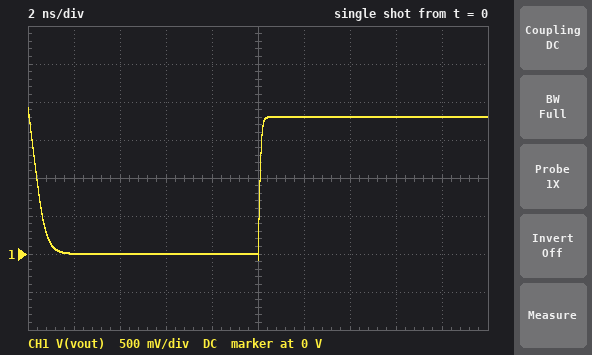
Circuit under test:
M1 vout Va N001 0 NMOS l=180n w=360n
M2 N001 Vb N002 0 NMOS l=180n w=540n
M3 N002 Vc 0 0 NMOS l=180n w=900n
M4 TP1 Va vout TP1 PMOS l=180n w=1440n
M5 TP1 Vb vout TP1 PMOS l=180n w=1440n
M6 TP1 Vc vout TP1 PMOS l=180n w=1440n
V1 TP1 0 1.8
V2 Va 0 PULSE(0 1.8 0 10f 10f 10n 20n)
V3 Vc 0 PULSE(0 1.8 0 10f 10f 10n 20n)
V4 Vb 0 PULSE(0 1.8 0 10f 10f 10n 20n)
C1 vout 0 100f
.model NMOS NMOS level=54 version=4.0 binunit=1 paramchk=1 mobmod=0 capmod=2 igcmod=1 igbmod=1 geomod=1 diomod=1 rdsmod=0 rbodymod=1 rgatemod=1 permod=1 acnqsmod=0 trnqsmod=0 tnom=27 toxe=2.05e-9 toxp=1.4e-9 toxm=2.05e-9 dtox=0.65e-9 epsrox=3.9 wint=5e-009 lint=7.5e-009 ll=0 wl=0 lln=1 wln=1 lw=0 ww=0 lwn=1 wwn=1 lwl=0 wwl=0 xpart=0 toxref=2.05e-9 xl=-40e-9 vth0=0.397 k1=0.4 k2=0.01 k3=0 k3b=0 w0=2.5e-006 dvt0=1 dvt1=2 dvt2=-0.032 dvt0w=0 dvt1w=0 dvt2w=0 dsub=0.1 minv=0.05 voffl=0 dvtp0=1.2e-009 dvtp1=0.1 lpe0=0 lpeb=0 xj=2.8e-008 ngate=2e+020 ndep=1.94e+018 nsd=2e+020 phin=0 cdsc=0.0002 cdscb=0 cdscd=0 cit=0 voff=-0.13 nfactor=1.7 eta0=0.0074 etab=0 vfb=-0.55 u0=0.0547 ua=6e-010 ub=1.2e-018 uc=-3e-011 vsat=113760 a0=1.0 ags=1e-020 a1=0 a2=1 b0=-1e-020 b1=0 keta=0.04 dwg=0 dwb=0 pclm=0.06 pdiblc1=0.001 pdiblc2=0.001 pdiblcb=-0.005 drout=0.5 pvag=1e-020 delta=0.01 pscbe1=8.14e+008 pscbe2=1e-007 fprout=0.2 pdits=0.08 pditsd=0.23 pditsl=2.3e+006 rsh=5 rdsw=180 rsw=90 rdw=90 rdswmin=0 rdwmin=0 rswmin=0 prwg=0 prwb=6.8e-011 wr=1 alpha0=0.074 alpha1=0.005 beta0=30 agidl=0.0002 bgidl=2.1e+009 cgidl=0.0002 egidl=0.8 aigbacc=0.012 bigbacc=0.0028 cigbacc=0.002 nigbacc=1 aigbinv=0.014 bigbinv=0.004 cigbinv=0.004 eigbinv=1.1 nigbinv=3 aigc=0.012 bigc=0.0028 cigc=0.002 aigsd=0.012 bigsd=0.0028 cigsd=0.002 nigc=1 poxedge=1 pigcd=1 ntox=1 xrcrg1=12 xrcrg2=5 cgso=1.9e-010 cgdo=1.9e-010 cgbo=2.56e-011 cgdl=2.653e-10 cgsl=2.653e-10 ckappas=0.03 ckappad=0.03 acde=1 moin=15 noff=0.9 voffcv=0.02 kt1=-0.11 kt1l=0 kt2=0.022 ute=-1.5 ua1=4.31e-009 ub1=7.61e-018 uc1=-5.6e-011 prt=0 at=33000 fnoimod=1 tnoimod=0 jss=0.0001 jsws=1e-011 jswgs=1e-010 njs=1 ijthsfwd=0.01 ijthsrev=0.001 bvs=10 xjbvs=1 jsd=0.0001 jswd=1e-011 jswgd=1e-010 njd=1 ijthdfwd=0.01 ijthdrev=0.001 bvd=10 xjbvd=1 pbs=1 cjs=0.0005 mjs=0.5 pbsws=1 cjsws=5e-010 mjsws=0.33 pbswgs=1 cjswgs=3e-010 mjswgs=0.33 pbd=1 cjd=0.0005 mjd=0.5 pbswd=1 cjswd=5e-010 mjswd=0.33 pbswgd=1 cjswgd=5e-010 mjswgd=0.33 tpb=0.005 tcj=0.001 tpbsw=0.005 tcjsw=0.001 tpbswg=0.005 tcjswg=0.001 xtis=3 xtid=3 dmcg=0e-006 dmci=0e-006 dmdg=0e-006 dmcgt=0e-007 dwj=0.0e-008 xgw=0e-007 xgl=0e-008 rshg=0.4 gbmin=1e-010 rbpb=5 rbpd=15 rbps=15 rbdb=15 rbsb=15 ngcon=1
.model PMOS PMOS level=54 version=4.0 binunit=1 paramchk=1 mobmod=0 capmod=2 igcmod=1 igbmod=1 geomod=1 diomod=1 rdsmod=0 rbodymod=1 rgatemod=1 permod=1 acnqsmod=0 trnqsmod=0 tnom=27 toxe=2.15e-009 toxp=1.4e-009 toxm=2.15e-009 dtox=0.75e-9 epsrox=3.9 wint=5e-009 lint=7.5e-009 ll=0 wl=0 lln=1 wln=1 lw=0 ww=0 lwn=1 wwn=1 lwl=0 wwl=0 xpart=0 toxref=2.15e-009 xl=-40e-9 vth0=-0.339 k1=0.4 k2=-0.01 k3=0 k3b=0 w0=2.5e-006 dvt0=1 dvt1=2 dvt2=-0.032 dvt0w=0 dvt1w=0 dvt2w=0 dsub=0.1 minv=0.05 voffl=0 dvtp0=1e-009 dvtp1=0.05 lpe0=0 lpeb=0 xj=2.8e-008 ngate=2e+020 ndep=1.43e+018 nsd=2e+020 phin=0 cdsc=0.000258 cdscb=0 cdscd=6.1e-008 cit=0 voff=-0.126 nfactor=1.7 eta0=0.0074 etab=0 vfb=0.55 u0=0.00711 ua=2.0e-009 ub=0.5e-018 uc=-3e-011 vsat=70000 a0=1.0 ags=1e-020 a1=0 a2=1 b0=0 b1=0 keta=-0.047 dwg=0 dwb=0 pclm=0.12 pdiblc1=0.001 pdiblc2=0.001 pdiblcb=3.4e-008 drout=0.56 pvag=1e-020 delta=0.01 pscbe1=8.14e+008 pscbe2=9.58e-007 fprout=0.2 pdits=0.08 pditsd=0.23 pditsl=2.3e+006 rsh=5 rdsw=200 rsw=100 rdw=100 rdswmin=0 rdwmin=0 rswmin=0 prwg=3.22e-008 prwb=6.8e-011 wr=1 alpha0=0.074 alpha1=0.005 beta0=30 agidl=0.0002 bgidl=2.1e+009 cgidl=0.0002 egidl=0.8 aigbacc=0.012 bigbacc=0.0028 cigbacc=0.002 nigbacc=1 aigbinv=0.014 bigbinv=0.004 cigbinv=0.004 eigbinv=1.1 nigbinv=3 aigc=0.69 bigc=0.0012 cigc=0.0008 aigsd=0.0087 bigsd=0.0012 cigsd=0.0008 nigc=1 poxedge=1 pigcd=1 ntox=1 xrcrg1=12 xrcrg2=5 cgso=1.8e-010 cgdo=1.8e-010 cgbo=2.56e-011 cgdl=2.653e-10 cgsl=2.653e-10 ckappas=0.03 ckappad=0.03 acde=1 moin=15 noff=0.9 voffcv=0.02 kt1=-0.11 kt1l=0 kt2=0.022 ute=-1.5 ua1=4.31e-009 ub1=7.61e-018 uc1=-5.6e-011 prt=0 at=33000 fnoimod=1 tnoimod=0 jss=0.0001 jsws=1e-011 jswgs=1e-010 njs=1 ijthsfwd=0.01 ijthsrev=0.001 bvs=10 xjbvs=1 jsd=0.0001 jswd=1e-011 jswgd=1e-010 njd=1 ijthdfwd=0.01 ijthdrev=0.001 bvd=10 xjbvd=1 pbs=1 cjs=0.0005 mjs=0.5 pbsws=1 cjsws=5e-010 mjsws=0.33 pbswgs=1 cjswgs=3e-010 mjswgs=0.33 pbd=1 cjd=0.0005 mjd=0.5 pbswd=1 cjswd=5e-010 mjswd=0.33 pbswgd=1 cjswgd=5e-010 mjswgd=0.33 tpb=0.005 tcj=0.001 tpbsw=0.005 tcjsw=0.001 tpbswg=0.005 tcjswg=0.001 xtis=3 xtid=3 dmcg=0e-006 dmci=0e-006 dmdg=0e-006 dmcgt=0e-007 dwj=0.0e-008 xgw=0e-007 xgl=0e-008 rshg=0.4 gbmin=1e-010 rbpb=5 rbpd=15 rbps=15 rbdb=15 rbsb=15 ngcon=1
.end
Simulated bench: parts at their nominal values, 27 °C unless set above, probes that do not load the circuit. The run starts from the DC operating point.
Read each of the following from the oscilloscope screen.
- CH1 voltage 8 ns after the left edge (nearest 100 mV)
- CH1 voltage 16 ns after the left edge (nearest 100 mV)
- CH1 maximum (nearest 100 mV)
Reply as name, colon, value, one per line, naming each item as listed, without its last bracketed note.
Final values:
CH1 voltage 8 ns after the left edge: 0 V
CH1 voltage 16 ns after the left edge: 1.8 V
CH1 maximum: 1.9 V
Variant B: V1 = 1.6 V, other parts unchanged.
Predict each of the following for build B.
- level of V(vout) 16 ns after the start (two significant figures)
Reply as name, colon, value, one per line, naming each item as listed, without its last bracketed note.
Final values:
level of V(vout) 16 ns after the start: 1.6 V
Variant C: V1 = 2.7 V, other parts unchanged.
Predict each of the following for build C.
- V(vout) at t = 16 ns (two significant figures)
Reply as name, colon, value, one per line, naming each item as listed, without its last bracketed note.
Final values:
V(vout) at t = 16 ns: 2.7 V
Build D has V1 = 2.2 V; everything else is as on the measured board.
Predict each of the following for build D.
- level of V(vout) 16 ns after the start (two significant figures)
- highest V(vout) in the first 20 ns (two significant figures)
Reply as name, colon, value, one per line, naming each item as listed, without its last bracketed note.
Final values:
level of V(vout) 16 ns after the start: 2.2 V
highest V(vout) in the first 20 ns: 2.3 V
